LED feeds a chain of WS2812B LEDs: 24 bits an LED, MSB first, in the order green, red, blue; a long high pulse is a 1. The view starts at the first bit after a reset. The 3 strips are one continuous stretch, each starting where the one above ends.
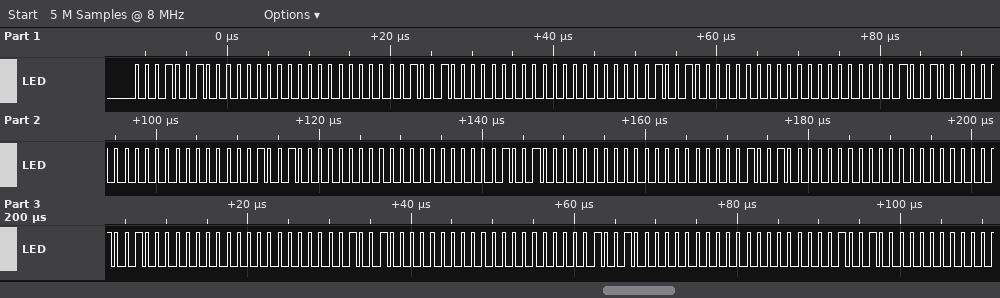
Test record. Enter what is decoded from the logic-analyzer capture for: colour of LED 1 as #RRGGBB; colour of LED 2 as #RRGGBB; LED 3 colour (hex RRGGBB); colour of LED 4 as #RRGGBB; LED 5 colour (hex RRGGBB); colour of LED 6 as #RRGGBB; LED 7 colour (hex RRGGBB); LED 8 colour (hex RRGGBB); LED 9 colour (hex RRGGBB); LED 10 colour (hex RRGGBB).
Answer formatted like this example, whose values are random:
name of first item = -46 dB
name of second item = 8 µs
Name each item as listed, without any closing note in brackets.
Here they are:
colour of LED 1 as #RRGGBB = #001200
colour of LED 2 as #RRGGBB = #001200
LED 3 colour = #001200
colour of LED 4 as #RRGGBB = #001200
LED 5 colour = #001200
colour of LED 6 as #RRGGBB = #001200
LED 7 colour = #001200
LED 8 colour = #001200
LED 9 colour = #001200
LED 10 colour = #001200
